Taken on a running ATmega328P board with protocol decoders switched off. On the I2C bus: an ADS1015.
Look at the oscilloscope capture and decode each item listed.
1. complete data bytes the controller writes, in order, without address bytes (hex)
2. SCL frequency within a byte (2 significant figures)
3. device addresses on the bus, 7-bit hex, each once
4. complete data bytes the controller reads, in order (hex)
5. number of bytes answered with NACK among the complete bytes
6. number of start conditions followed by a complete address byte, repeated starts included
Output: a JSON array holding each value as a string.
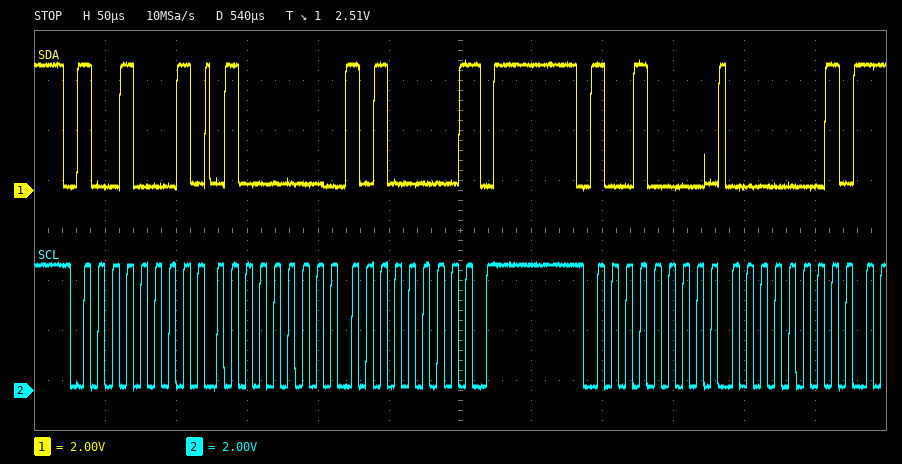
["01", "100 kHz", "0x48", "40 A0", "1", "2"]
